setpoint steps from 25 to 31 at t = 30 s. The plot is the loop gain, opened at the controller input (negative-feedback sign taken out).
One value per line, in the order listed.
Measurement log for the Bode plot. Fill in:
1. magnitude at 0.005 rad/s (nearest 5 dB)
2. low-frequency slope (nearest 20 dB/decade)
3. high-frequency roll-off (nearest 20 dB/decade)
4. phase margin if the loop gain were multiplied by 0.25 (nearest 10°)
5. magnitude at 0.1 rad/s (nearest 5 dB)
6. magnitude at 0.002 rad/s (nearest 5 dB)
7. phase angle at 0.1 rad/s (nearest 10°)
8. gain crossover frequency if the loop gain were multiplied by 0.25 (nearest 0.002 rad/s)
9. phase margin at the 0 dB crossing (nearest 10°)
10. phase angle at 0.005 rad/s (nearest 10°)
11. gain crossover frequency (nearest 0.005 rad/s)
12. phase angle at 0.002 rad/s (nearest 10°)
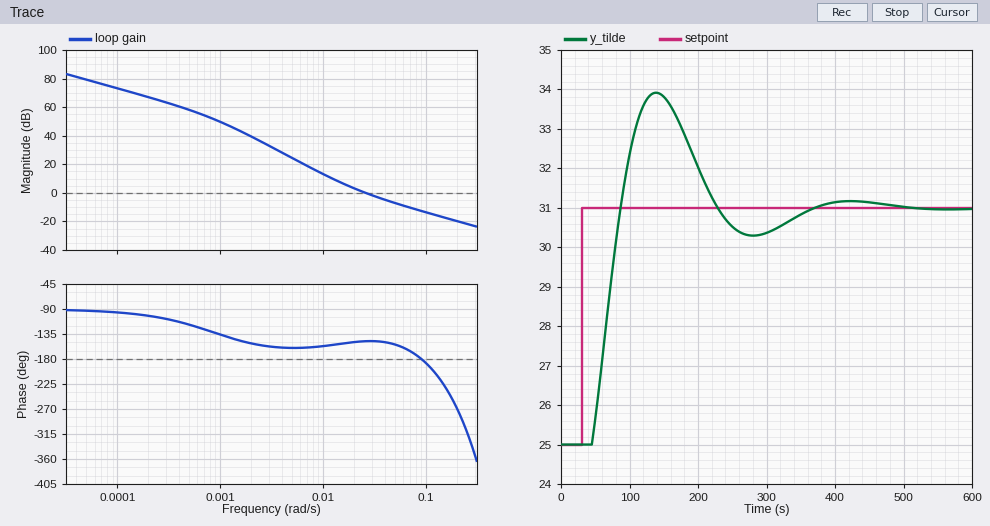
25 dB
-20 dB/decade
-20 dB/decade
20°
-15 dB
40 dB
-190°
0.010 rad/s
30°
-160°
0.025 rad/s
-150°
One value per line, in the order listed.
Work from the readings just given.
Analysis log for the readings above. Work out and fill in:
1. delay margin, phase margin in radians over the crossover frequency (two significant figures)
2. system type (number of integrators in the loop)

21 s
1
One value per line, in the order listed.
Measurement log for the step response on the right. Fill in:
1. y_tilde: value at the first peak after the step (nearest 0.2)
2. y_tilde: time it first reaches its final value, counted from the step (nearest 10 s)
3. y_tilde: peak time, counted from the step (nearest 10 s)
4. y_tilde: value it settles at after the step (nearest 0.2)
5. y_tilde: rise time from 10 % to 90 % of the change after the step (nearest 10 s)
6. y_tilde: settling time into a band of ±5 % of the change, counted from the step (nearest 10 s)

34.0
60 s
110 s
31.0
30 s
310 s
